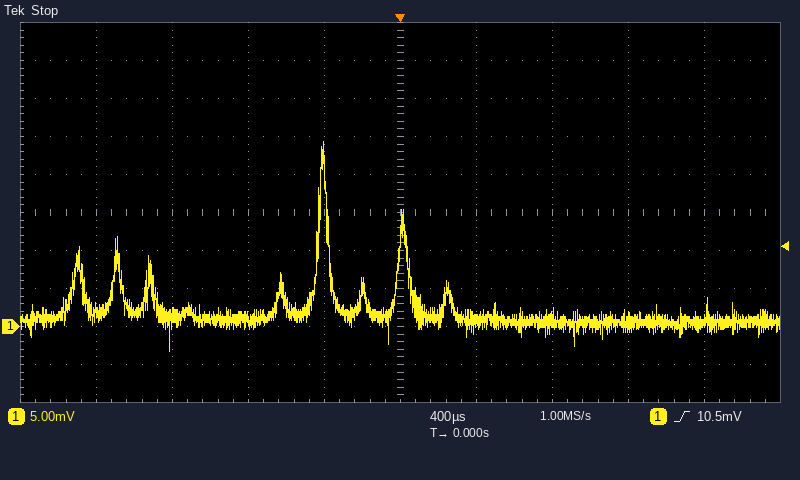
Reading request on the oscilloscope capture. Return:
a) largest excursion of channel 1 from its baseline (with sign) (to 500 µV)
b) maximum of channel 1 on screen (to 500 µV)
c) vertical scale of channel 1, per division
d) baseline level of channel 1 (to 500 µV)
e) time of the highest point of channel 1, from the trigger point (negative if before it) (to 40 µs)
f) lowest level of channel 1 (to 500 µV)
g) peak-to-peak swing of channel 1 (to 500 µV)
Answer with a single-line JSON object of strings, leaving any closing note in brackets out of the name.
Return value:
{"largest excursion of channel 1 from its baseline (with sign)": "+23.5 mV", "maximum of channel 1 on screen": "24.5 mV", "vertical scale of channel 1, per division": "5 mV", "baseline level of channel 1": "1.0 mV", "time of the highest point of channel 1, from the trigger point (negative if before it)": "-400 µs", "lowest level of channel 1": "-3.0 mV", "peak-to-peak swing of channel 1": "27.5 mV"}
